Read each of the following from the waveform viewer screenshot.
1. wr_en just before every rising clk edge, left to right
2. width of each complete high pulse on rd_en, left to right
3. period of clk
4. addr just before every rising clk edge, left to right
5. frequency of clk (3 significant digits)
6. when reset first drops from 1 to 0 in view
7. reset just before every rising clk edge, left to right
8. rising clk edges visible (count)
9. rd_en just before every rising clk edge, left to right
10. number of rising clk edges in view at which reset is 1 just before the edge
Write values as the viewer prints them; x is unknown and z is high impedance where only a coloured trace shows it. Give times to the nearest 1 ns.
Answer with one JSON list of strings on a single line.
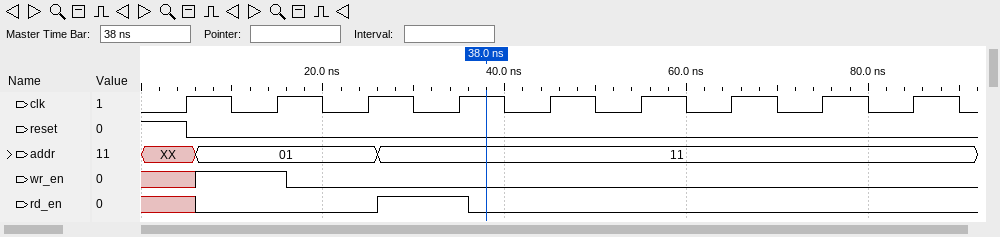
["x 1 0 0 0 0 0 0 0", "10 ns", "10 ns", "XX, 01, 01, 11, 11, 11, 11, 11, 11", "100 MHz", "5 ns", "1 0 0 0 0 0 0 0 0", "9", "x 0 0 1 0 0 0 0 0", "1"]
